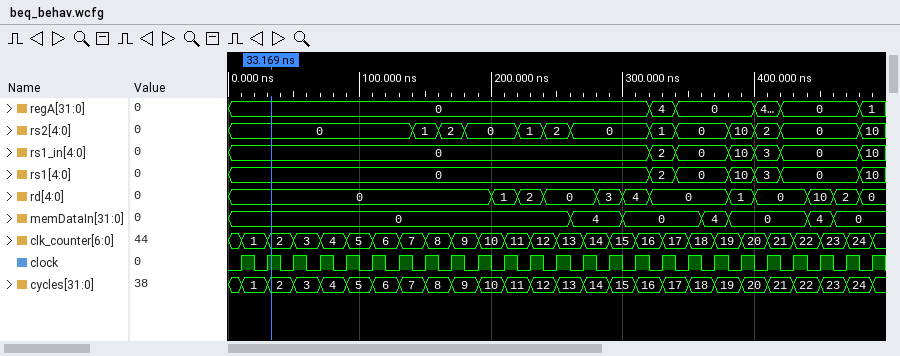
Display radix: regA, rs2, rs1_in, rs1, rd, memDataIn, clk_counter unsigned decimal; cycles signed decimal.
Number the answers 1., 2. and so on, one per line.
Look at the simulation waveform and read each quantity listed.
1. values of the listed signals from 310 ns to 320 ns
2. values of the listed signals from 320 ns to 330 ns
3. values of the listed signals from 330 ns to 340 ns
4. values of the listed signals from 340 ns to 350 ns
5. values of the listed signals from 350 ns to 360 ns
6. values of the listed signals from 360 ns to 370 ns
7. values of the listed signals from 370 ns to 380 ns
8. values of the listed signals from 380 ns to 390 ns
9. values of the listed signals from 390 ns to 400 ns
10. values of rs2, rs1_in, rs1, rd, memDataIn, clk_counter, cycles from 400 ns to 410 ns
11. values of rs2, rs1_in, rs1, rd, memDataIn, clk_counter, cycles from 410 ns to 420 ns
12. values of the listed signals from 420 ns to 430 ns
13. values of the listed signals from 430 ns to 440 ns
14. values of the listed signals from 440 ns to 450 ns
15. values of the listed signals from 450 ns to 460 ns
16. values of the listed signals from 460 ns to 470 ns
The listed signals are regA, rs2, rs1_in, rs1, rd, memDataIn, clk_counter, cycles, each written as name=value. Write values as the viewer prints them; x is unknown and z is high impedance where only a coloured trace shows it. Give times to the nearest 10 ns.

1. regA=0, rs2=0, rs1_in=0, rs1=0, rd=4, memDataIn=0, clk_counter=16, cycles=16
2. regA=4, rs2=1, rs1_in=2, rs1=2, rd=0, memDataIn=0, clk_counter=16, cycles=16
3. regA=4, rs2=1, rs1_in=2, rs1=2, rd=0, memDataIn=0, clk_counter=17, cycles=17
4. regA=0, rs2=0, rs1_in=0, rs1=0, rd=0, memDataIn=0, clk_counter=17, cycles=17
5. regA=0, rs2=0, rs1_in=0, rs1=0, rd=0, memDataIn=0, clk_counter=18, cycles=18
6. regA=0, rs2=0, rs1_in=0, rs1=0, rd=0, memDataIn=4, clk_counter=18, cycles=18
7. regA=0, rs2=0, rs1_in=0, rs1=0, rd=0, memDataIn=4, clk_counter=19, cycles=19
8. regA=0, rs2=10, rs1_in=10, rs1=10, rd=1, memDataIn=0, clk_counter=19, cycles=19
9. regA=0, rs2=10, rs1_in=10, rs1=10, rd=1, memDataIn=0, clk_counter=20, cycles=20
10. rs2=2, rs1_in=3, rs1=3, rd=0, memDataIn=0, clk_counter=20, cycles=20
11. rs2=2, rs1_in=3, rs1=3, rd=0, memDataIn=0, clk_counter=21, cycles=21
12. regA=0, rs2=0, rs1_in=0, rs1=0, rd=0, memDataIn=0, clk_counter=21, cycles=21
13. regA=0, rs2=0, rs1_in=0, rs1=0, rd=0, memDataIn=0, clk_counter=22, cycles=22
14. regA=0, rs2=0, rs1_in=0, rs1=0, rd=10, memDataIn=4, clk_counter=22, cycles=22
15. regA=0, rs2=0, rs1_in=0, rs1=0, rd=10, memDataIn=4, clk_counter=23, cycles=23
16. regA=0, rs2=0, rs1_in=0, rs1=0, rd=2, memDataIn=0, clk_counter=23, cycles=23
